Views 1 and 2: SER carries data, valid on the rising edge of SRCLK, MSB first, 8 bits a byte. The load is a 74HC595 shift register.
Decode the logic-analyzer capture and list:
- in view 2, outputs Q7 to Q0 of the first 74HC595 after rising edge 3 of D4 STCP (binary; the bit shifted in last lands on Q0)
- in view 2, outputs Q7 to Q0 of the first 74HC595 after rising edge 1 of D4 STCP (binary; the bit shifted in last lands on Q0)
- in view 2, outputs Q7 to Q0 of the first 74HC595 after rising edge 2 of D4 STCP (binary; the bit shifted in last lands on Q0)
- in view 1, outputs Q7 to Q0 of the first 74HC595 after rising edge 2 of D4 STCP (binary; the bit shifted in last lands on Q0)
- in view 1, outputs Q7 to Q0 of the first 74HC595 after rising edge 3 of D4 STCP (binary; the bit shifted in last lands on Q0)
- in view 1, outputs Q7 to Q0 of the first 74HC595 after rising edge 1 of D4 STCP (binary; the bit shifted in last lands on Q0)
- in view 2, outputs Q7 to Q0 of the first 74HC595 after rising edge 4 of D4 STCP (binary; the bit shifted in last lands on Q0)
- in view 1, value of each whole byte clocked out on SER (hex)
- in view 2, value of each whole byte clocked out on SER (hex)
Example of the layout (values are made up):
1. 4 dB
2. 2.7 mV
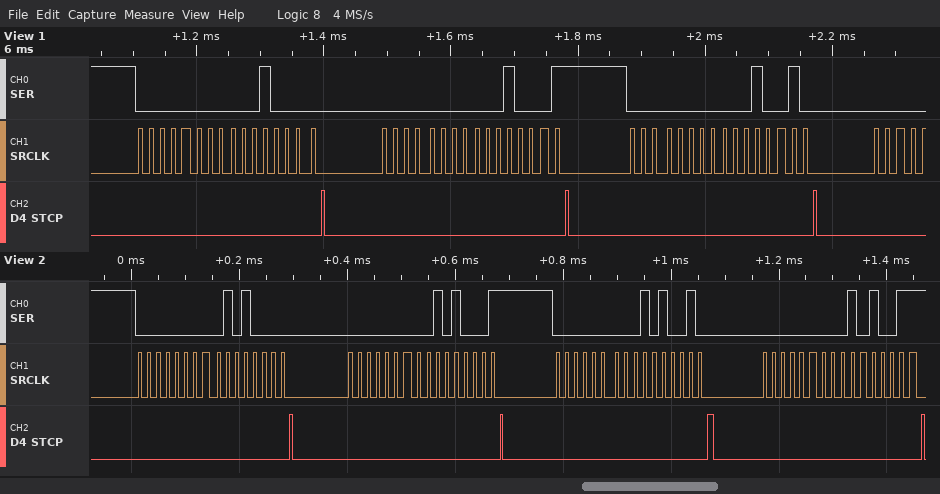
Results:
1. 01010010
2. 01010000
3. 01010001
4. 00010001
5. 00010010
6. 00010000
7. 01010011
8. 00 10 00 11 00 12
9. 00 50 00 51 00 52 00 53
